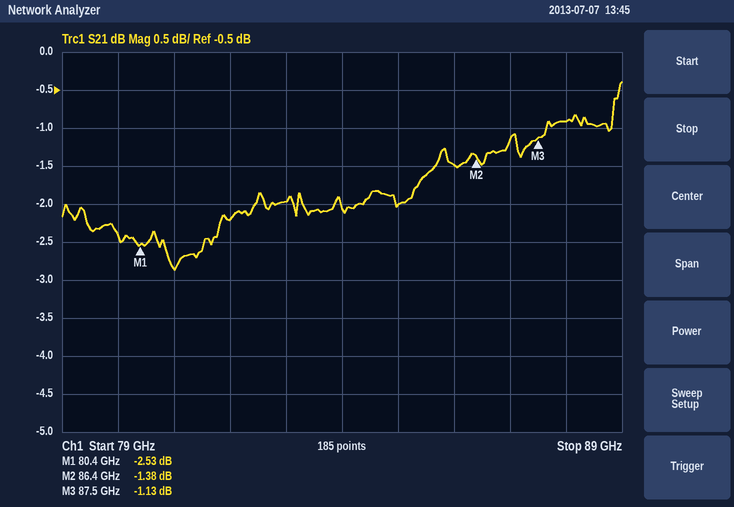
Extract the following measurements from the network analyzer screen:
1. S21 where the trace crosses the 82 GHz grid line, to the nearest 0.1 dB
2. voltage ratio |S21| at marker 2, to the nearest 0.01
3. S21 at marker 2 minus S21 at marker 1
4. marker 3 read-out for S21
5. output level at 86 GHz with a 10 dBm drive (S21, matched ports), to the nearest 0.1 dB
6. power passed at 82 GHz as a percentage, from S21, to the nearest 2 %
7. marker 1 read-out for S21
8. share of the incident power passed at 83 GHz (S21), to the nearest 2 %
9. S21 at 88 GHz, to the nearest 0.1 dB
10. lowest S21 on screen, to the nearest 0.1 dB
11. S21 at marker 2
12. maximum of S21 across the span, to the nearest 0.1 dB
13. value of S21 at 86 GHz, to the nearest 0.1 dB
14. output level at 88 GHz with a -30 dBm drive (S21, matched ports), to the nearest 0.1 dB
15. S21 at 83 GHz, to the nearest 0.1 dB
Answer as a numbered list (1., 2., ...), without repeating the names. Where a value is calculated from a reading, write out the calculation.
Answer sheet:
1. -2.2 dB
2. 10^(-1.38/20) ≈ 0.85
3. -1.38 − (-2.53) = 1.15 dB
4. -1.13 dB
5. 10 dBm + (-1.5 dB) = 8.5 dBm
6. 10^(-2.2/10) ≈ 60 %
7. -2.53 dB
8. 10^(-2/10) ≈ 63.1 %, so 64 % to the nearest 2 %
9. -0.9 dB
10. -2.9 dB
11. -1.38 dB
12. -0.4 dB
13. -1.5 dB
14. -30 dBm + (-0.9 dB) = -30.9 dBm
15. -2.0 dB
